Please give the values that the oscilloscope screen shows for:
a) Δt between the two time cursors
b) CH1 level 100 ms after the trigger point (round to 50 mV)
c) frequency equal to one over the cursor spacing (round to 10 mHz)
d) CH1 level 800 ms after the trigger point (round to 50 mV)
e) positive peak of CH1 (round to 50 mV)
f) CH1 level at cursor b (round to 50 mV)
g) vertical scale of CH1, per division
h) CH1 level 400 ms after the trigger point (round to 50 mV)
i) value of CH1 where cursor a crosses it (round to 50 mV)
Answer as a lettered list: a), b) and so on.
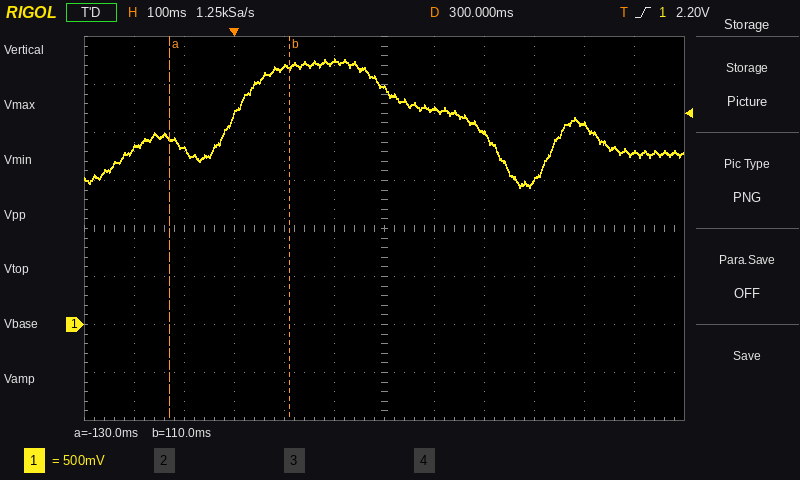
a) 240 ms
b) 2.70 V
c) 4.17 Hz
d) 1.80 V
e) 2.75 V
f) 2.70 V
g) 500 mV
h) 2.25 V
i) 1.95 V
